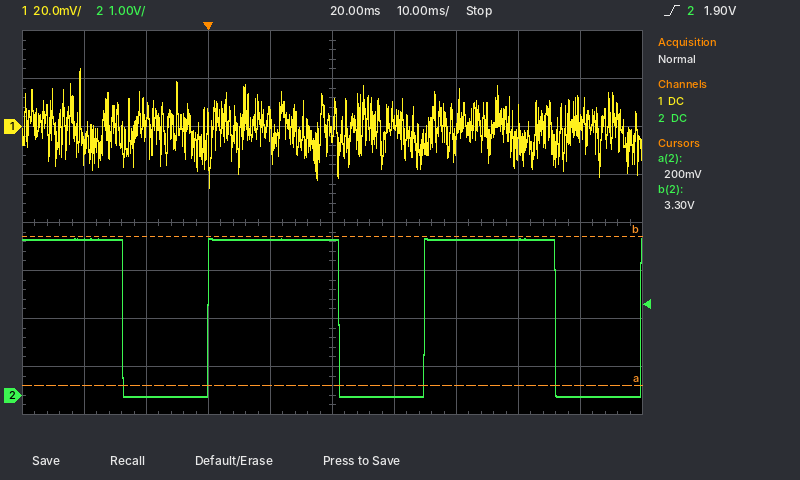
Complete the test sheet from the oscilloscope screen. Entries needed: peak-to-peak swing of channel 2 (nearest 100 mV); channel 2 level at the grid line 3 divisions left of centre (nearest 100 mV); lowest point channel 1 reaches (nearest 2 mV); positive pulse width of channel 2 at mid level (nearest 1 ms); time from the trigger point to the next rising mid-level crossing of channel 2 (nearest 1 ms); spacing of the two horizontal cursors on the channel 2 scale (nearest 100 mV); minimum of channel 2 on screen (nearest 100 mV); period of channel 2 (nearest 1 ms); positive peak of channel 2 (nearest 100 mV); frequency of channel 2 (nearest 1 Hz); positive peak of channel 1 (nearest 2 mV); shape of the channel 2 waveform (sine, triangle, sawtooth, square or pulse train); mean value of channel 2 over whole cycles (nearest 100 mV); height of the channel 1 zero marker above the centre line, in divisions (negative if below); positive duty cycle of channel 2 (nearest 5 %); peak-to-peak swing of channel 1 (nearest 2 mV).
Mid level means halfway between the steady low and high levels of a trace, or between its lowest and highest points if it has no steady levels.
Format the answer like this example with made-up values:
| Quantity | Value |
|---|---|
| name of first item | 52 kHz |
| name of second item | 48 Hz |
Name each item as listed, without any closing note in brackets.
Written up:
| Quantity | Value |
|---|---|
| peak-to-peak swing of channel 2 | 3.3 V |
| channel 2 level at the grid line 3 divisions left of centre | 0.0 V |
| lowest point channel 1 reaches | -26 mV |
| positive pulse width of channel 2 at mid level | 21 ms |
| time from the trigger point to the next rising mid-level crossing of channel 2 | 35 ms |
| spacing of the two horizontal cursors on the channel 2 scale | 3.1 V |
| minimum of channel 2 on screen | 0.0 V |
| period of channel 2 | 35 ms |
| positive peak of channel 2 | 3.3 V |
| frequency of channel 2 | 29 Hz |
| positive peak of channel 1 | 24 mV |
| shape of the channel 2 waveform | pulse train |
| mean value of channel 2 over whole cycles | 2.0 V |
| height of the channel 1 zero marker above the centre line, in divisions | +2.0 div |
| positive duty cycle of channel 2 | 60 % |
| peak-to-peak swing of channel 1 | 50 mV |
